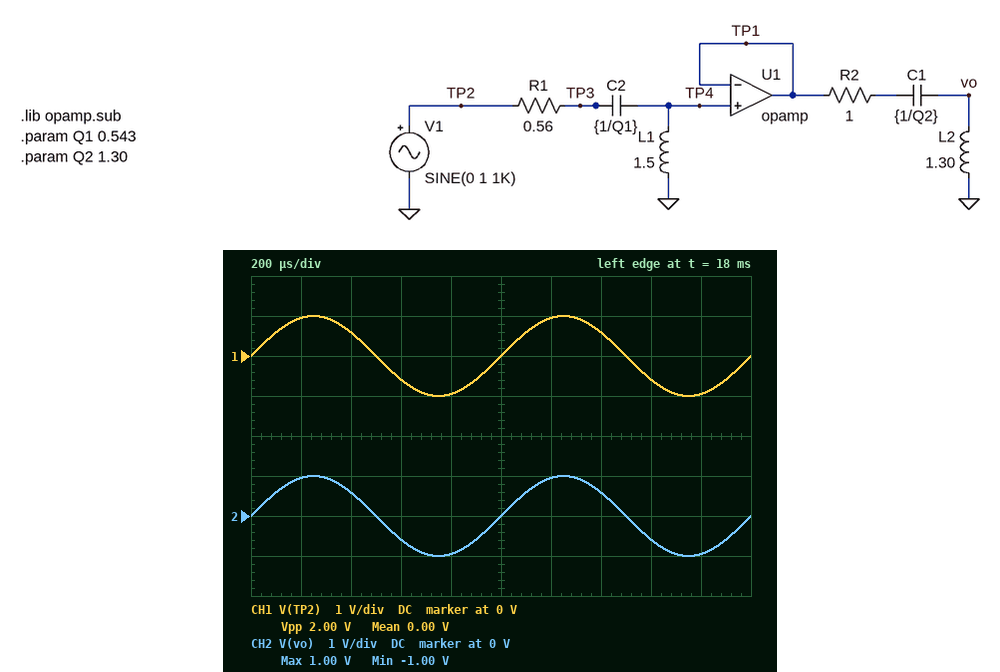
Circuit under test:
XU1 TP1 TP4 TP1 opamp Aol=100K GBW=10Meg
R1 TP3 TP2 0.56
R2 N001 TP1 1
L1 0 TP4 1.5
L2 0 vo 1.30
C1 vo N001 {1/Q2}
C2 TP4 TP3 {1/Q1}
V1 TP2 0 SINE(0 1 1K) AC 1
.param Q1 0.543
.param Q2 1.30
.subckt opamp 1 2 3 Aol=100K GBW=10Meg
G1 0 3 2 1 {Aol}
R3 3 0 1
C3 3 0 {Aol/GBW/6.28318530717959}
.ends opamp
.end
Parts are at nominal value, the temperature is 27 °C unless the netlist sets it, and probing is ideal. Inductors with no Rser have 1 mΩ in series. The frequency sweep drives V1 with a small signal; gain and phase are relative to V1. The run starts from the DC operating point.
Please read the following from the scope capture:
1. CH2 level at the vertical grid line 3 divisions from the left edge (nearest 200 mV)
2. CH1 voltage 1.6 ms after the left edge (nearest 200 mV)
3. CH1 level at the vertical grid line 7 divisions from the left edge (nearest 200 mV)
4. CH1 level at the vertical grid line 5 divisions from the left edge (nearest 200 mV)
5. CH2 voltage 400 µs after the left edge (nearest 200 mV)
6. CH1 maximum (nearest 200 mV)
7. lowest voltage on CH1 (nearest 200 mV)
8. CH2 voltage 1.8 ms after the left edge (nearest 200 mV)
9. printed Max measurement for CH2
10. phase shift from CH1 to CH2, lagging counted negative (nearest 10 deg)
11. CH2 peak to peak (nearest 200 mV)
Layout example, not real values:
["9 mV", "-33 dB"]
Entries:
["-600 mV", "-600 mV", "600 mV", "0 V", "600 mV", "1.0 V", "-1.0 V", "-1.0 V", "1.00 V", "0 deg", "2.0 V"]
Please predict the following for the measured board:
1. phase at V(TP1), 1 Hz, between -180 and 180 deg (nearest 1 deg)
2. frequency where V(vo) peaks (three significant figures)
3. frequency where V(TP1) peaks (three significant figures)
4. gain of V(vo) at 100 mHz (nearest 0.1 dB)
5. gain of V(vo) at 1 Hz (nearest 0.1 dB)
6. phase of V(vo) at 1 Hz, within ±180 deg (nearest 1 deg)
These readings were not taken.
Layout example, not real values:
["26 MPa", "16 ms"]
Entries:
["3 deg", "171 mHz", "107 mHz", "-1.4 dB", "0.2 dB", "11 deg"]
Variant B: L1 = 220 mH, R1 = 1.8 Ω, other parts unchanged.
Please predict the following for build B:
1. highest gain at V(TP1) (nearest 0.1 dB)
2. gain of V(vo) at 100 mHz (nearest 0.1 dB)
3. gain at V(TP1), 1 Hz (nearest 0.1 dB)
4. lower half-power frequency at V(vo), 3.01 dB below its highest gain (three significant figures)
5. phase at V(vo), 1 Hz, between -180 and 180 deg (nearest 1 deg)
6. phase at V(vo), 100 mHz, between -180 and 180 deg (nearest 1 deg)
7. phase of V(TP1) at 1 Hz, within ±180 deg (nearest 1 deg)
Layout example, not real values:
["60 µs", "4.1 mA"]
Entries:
["0 dB", "-28.8 dB", "-4.1 dB", "1.23 Hz", "61 deg", "-107 deg", "54 deg"]
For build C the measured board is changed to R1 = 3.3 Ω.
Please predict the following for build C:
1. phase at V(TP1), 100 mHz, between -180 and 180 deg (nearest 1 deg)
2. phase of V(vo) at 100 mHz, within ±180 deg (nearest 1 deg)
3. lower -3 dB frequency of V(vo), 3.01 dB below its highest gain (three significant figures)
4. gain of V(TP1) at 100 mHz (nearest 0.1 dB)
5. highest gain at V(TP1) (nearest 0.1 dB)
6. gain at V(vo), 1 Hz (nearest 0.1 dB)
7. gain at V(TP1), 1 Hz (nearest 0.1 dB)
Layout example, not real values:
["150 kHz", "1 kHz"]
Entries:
["89 deg", "-130 deg", "190 mHz", "-10.9 dB", "0 dB", "-0.3 dB", "-0.4 dB"]
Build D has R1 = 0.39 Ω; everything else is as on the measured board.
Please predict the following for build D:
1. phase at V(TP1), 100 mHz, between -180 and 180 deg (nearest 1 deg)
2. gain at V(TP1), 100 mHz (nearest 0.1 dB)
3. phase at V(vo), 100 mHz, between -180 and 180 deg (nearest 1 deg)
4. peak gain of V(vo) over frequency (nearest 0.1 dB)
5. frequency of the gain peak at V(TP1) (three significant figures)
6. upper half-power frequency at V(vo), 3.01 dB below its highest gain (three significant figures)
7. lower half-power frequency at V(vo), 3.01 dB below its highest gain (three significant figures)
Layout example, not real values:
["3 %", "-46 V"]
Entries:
["79 deg", "7.5 dB", "-140 deg", "5.5 dB", "101 mHz", "298 mHz", "105 mHz"]
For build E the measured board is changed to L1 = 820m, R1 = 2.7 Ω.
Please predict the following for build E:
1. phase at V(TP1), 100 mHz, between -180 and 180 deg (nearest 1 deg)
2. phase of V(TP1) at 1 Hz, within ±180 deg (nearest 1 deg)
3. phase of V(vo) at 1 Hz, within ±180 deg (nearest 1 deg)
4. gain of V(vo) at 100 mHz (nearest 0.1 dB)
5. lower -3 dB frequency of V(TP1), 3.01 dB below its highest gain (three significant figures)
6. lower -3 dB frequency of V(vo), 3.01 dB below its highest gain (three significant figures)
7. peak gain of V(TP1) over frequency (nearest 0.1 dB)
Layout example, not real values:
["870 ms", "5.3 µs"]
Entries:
["97 deg", "28 deg", "35 deg", "-20.3 dB", "492 mHz", "405 mHz", "0 dB"]
